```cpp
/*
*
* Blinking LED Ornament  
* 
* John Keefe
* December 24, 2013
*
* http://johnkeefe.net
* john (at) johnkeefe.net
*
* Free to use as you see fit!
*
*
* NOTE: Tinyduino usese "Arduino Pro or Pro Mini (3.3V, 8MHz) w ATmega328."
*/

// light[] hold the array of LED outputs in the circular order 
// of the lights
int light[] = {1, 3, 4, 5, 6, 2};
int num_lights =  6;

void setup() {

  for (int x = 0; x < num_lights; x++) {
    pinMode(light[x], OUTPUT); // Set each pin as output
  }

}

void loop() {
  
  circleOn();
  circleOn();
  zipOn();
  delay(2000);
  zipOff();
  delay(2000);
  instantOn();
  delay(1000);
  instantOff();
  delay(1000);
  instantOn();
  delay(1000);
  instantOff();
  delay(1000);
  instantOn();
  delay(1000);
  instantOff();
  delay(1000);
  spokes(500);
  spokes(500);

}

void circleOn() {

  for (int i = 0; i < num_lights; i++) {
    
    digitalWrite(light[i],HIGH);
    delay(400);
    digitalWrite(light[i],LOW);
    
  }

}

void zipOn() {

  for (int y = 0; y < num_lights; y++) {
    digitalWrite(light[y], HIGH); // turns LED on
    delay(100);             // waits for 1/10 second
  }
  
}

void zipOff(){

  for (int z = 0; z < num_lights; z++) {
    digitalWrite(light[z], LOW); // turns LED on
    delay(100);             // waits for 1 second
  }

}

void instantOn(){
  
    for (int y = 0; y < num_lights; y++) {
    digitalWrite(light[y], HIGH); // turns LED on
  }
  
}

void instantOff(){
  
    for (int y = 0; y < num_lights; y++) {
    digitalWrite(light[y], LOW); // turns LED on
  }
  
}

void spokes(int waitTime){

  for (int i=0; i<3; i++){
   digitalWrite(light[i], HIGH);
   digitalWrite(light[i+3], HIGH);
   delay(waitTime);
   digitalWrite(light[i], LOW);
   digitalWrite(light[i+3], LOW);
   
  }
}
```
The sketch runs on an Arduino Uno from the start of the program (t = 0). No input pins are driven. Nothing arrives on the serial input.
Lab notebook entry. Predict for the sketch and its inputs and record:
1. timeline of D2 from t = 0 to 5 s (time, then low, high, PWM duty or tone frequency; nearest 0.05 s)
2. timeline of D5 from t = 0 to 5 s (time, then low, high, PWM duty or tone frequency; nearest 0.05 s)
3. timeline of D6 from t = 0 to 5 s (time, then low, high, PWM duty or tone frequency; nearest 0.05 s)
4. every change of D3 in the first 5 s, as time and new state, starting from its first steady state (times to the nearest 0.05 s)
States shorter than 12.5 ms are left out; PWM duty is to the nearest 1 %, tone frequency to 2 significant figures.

0 s low; 2 s high; 2.4 s low; 4.4 s high; 4.8 s low
0 s low; 1.2 s high; 1.6 s low; 3.6 s high; 4 s low
0 s low; 1.6 s high; 2 s low; 4 s high; 4.4 s low
0 s low; 0.4 s high; 0.8 s low; 2.8 s high; 3.2 s low; 4.9 s high
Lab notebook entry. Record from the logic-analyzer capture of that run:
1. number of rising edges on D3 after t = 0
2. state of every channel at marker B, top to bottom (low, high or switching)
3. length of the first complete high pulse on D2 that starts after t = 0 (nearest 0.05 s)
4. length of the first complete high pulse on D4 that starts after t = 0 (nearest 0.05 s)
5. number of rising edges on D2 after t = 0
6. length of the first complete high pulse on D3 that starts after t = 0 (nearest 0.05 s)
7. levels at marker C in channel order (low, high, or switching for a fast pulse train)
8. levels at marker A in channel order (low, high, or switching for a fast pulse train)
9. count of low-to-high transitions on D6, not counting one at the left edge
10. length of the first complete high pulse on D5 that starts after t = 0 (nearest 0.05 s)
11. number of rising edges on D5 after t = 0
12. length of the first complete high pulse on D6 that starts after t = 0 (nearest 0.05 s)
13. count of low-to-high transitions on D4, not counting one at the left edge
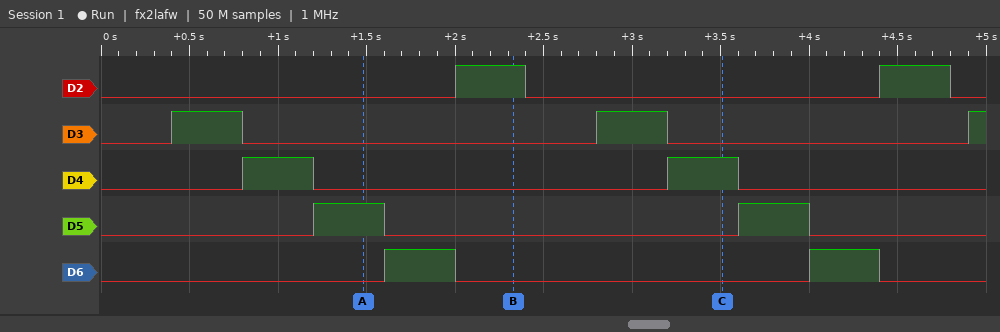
3
D2 high, D3 low, D4 low, D5 low, D6 low
0.40 s
0.40 s
2
0.40 s
D2 low, D3 low, D4 high, D5 low, D6 low
D2 low, D3 low, D4 low, D5 high, D6 low
2
0.40 s
2
0.40 s
2
